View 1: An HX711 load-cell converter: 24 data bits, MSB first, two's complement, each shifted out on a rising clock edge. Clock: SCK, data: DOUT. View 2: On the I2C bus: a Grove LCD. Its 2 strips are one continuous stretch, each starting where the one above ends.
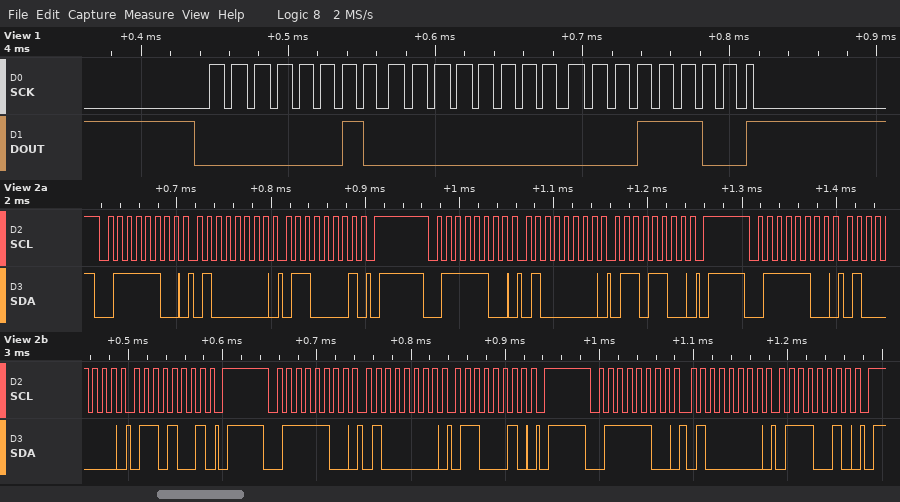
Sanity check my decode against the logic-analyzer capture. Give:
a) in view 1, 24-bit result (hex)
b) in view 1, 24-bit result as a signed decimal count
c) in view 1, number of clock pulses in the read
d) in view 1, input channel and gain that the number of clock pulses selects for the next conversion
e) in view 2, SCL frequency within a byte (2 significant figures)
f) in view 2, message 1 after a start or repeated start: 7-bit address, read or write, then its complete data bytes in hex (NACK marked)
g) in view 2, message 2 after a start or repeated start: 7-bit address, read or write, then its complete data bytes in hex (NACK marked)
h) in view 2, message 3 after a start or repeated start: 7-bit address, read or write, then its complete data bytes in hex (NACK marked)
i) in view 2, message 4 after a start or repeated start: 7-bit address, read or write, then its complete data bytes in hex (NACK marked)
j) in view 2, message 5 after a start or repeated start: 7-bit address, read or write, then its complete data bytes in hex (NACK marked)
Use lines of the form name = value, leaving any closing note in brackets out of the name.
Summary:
in view 1, 24-bit result = 0x02001C
in view 1, 24-bit result as a signed decimal count = 131100
in view 1, number of clock pulses in the read = 25
in view 1, input channel and gain that the number of clock pulses selects for the next conversion = channel A, gain 128
in view 2, SCL frequency within a byte = 100 kHz
in view 2, message 1 after a start or repeated start: 7-bit address, read or write, then its complete data bytes in hex = 0x3E write: 40 61
in view 2, message 2 after a start or repeated start: 7-bit address, read or write, then its complete data bytes in hex = 0x3E write: 40 6C
in view 2, message 3 after a start or repeated start: 7-bit address, read or write, then its complete data bytes in hex = 0x3E write: 40 69
in view 2, message 4 after a start or repeated start: 7-bit address, read or write, then its complete data bytes in hex = 0x3E write: 40 62
in view 2, message 5 after a start or repeated start: 7-bit address, read or write, then its complete data bytes in hex = 0x3E write: 40 72
